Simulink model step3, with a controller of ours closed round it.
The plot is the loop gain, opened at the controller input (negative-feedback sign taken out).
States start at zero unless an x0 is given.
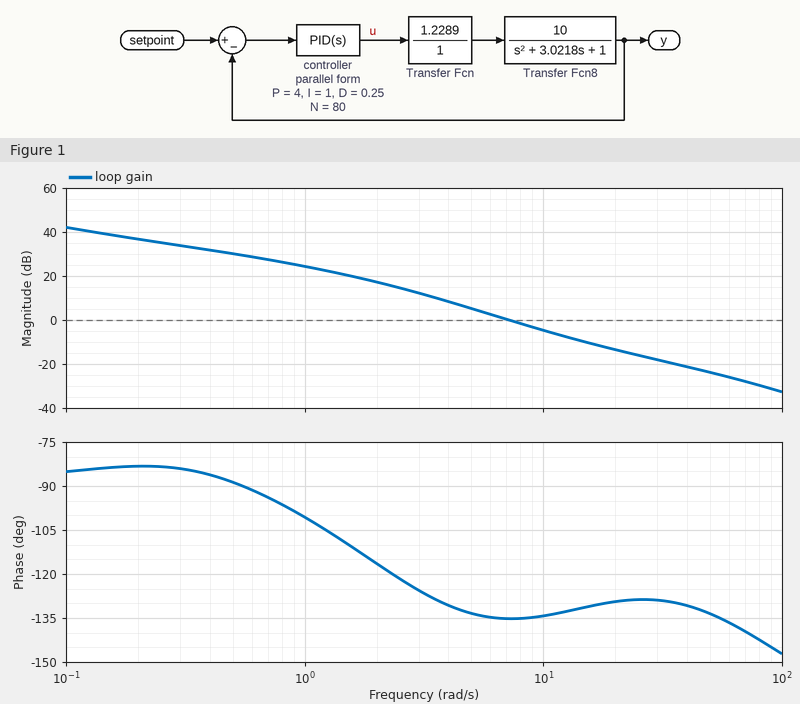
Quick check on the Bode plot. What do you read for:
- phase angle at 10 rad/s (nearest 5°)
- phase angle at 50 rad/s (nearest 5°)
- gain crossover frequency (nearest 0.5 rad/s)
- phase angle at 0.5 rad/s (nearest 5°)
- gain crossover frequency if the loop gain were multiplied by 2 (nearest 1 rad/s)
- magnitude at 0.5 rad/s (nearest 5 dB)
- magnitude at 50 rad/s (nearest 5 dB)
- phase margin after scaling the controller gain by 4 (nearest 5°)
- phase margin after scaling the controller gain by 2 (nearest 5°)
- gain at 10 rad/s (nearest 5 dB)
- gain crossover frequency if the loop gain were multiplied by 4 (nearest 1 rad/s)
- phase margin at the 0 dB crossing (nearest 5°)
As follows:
-135°
-135°
7.0 rad/s
-90°
11 rad/s
30 dB
-25 dB
50°
45°
-5 dB
18 rad/s
45°
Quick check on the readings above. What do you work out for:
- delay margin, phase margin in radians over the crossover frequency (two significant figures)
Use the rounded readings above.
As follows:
0.11 s
